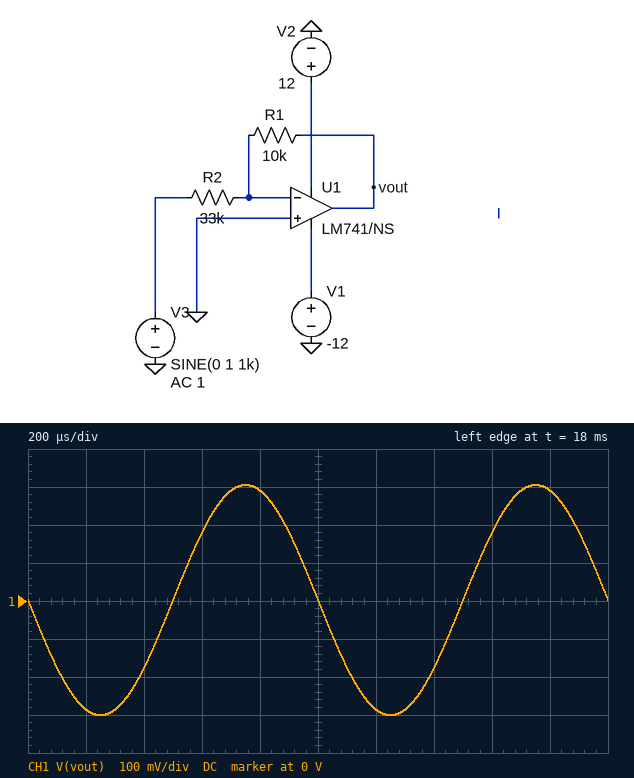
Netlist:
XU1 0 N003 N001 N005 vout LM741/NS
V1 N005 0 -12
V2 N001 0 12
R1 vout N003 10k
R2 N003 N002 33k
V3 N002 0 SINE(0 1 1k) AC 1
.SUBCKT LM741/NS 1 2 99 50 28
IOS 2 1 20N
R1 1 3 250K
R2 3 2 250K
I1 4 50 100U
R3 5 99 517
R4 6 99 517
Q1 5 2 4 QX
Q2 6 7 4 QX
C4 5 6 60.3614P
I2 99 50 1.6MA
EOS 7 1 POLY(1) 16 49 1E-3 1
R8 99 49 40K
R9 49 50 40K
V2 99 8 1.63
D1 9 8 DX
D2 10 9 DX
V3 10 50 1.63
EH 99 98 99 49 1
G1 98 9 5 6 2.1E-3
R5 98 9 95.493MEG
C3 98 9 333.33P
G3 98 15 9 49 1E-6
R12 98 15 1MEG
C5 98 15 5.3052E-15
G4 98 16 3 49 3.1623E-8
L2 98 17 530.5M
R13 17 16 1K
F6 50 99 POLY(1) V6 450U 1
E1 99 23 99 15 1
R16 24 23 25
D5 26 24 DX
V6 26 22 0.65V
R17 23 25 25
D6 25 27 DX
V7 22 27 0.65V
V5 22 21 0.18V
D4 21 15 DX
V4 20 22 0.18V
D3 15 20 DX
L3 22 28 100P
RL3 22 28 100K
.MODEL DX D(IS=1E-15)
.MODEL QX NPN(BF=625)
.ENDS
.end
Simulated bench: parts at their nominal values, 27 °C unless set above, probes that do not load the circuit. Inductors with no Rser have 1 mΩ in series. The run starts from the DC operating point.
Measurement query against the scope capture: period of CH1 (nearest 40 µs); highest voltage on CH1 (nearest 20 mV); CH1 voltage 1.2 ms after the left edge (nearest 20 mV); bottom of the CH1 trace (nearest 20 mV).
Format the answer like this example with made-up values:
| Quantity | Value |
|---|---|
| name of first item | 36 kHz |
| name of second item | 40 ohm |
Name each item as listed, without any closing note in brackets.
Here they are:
| Quantity | Value |
|---|---|
| period of CH1 | 1.00 ms |
| highest voltage on CH1 | 300 mV |
| CH1 voltage 1.2 ms after the left edge | -280 mV |
| bottom of the CH1 trace | -300 mV |
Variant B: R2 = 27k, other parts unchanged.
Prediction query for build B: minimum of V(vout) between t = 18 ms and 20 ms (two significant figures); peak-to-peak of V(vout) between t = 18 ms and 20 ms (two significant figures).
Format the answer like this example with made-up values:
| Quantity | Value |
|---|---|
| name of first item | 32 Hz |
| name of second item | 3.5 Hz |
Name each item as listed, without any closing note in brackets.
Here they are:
| Quantity | Value |
|---|---|
| minimum of V(vout) between t = 18 ms and 20 ms | -370 mV |
| peak-to-peak of V(vout) between t = 18 ms and 20 ms | 740 mV |
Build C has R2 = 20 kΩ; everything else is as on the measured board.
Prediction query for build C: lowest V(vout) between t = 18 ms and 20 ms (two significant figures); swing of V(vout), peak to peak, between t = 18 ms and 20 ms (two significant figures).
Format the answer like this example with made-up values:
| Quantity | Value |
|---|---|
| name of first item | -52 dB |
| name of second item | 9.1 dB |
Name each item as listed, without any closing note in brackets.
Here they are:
| Quantity | Value |
|---|---|
| lowest V(vout) between t = 18 ms and 20 ms | -500 mV |
| swing of V(vout), peak to peak, between t = 18 ms and 20 ms | 1.0 V |
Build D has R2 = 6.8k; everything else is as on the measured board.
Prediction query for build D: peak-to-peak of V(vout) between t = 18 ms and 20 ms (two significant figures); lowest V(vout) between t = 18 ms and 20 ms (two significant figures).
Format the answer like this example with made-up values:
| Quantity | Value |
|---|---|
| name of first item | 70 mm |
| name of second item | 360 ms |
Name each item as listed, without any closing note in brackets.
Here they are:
| Quantity | Value |
|---|---|
| peak-to-peak of V(vout) between t = 18 ms and 20 ms | 2.9 V |
| lowest V(vout) between t = 18 ms and 20 ms | -1.5 V |
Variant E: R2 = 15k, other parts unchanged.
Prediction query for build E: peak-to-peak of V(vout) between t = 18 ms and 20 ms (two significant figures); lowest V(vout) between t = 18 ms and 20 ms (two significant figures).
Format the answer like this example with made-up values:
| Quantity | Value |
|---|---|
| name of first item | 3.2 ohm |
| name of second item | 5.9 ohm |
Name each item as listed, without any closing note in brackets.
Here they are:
| Quantity | Value |
|---|---|
| peak-to-peak of V(vout) between t = 18 ms and 20 ms | 1.3 V |
| lowest V(vout) between t = 18 ms and 20 ms | -660 mV |
